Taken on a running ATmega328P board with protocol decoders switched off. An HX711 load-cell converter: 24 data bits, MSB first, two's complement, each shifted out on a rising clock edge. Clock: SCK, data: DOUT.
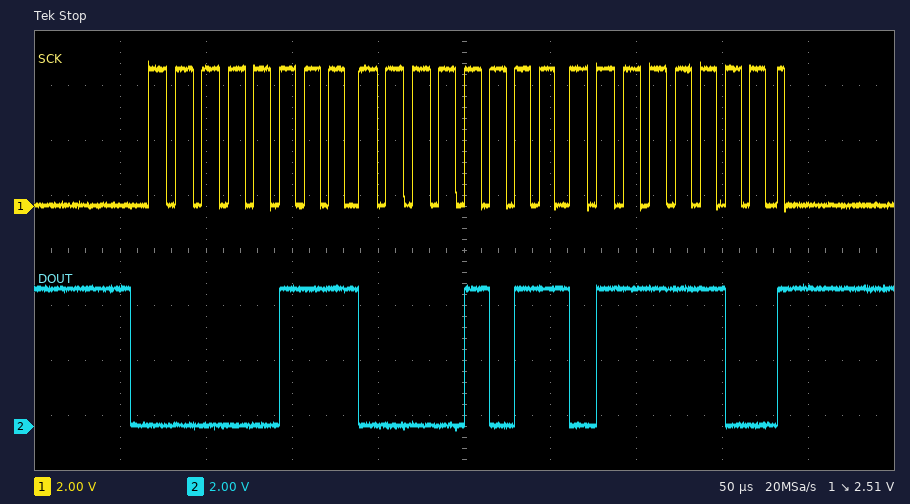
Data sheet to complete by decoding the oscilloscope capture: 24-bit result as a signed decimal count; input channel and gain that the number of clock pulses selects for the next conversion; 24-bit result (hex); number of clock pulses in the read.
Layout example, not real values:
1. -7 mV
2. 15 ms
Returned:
1. 461692
2. channel A, gain 128
3. 0x070B7C
4. 25
